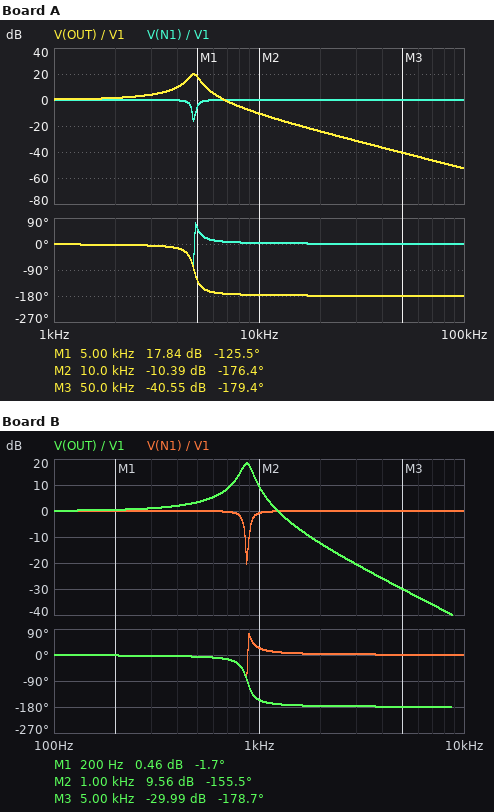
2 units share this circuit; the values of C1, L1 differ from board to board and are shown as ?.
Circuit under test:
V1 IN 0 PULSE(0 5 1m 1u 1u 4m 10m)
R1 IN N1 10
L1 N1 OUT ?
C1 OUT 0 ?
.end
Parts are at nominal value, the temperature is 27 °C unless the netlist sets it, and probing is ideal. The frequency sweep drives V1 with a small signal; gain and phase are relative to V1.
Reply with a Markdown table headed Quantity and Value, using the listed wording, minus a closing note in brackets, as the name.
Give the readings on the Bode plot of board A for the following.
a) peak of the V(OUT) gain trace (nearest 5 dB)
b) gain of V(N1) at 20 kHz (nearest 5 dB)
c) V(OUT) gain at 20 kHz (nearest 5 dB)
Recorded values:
| Quantity | Value |
|---|---|
| peak of the V(OUT) gain trace | 20 dB |
| gain of V(N1) at 20 kHz | 0 dB |
| V(OUT) gain at 20 kHz | -25 dB |
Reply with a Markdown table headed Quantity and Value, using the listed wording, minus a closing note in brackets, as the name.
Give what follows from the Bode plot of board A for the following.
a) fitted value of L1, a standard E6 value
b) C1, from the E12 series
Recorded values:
| Quantity | Value |
|---|---|
| fitted value of L1, a standard E6 value | 3.3 mH |
| C1, from the E12 series | 330 nF |
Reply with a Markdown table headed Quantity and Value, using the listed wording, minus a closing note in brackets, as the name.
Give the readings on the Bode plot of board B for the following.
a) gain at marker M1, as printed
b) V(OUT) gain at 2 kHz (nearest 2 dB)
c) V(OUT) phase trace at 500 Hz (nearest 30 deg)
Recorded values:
| Quantity | Value |
|---|---|
| gain at marker M1, as printed | 0.46 dB |
| V(OUT) gain at 2 kHz | -12 dB |
| V(OUT) phase trace at 500 Hz | 0 deg |
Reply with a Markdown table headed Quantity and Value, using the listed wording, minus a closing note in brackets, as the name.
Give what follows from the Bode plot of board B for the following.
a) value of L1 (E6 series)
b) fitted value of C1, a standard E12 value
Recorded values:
| Quantity | Value |
|---|---|
| value of L1 | 15 mH |
| fitted value of C1, a standard E12 value | 2.2 µF |
